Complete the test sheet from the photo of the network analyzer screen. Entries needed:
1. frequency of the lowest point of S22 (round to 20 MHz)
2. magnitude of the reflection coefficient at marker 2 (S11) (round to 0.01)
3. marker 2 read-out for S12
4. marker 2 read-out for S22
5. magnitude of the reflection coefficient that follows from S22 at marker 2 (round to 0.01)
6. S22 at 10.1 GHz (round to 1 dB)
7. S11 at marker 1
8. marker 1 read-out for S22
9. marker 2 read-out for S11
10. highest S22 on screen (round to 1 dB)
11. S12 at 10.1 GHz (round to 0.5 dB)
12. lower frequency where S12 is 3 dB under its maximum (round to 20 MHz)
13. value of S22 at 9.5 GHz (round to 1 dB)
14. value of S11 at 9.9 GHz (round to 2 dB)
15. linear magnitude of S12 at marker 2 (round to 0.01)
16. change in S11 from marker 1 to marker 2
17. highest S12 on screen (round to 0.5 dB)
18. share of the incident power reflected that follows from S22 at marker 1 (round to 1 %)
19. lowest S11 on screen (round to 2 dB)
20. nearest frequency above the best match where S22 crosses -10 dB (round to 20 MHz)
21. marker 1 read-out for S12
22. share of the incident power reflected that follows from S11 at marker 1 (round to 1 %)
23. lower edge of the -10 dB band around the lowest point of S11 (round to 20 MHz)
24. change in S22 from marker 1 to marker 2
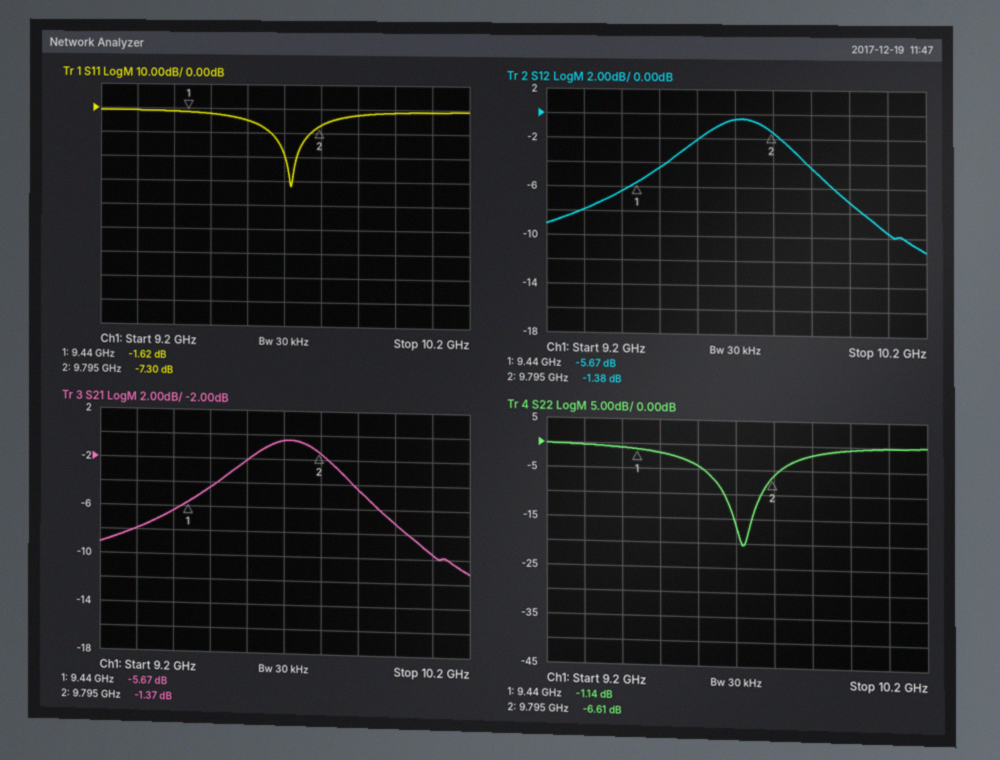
9.72 GHz
0.43
-1.38 dB
-6.61 dB
0.47
0 dB
-1.62 dB
-1.14 dB
-7.30 dB
0 dB
-9.5 dB
9.54 GHz
-2 dB
-2 dB
0.85
-5.68 dB
-0.5 dB
77 %
-32 dB
9.76 GHz
-5.67 dB
69 %
9.66 GHz
-5.47 dB
